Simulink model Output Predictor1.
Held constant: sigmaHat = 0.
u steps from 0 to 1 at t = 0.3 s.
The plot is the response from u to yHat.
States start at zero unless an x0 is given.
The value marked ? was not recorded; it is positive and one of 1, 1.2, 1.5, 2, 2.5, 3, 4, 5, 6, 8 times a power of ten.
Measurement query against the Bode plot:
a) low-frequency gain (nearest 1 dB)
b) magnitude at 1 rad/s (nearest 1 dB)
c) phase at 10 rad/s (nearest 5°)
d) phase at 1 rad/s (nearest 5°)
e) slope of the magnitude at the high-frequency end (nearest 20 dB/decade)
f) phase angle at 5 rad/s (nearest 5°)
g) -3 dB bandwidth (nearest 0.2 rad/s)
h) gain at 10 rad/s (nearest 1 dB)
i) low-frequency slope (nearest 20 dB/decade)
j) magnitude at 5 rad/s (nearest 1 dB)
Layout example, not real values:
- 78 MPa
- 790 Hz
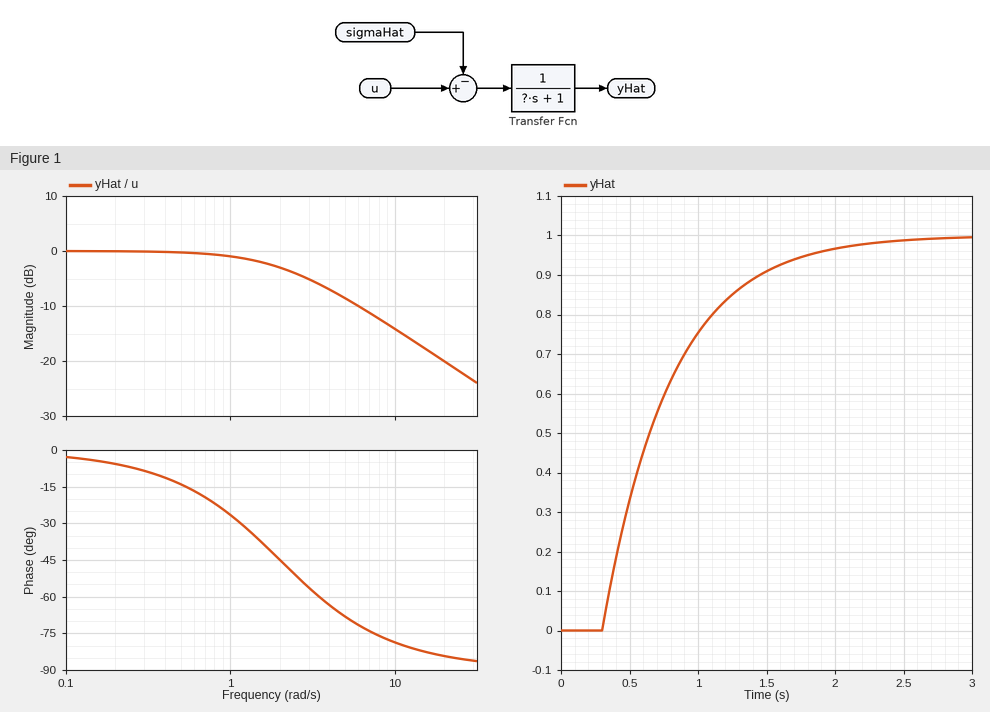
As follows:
- 0 dB
- -1 dB
- -80°
- -25°
- -20 dB/decade
- -70°
- 2.0 rad/s
- -14 dB
- 0 dB/decade
- -9 dB
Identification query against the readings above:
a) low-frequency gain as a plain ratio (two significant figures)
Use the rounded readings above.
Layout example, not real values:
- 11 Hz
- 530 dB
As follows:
- 1.0
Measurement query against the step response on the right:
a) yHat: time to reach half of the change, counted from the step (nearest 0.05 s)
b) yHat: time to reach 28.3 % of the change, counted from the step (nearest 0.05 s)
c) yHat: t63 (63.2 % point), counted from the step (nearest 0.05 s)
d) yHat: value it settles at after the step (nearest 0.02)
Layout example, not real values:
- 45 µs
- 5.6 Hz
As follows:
- 0.35 s
- 0.15 s
- 0.50 s
- 1.00
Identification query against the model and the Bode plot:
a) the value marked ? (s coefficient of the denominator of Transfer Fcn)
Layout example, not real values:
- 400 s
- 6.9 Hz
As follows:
- 0.5
